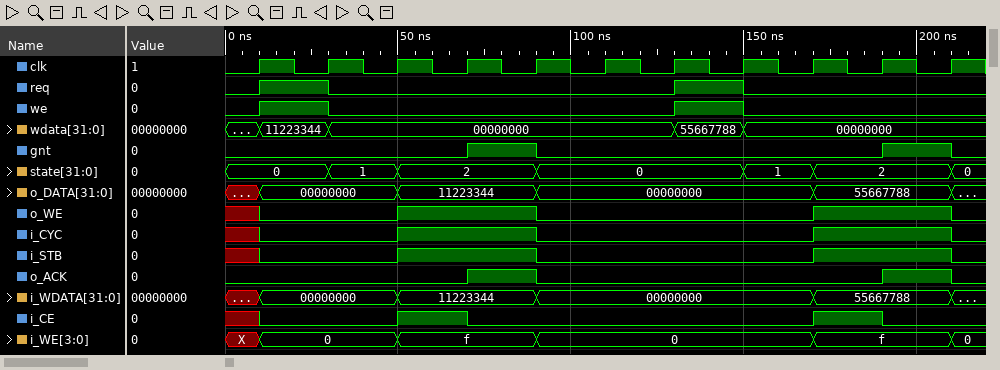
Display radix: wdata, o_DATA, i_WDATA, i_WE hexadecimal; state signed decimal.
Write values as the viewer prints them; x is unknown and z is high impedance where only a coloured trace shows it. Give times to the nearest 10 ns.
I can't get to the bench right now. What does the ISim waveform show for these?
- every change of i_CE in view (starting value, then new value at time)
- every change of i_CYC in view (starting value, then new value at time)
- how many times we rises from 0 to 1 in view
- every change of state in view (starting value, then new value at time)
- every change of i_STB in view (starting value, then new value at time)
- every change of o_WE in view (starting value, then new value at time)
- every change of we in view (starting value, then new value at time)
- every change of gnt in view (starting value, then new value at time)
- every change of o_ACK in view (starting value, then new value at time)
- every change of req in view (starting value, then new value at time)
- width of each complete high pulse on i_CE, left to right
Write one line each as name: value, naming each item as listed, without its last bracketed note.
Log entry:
every change of i_CE in view: x, 0 at 10 ns, 1 at 50 ns, 0 at 70 ns, 1 at 170 ns, 0 at 190 ns
every change of i_CYC in view: x, 0 at 10 ns, 1 at 50 ns, 0 at 90 ns, 1 at 170 ns, 0 at 210 ns
how many times we rises from 0 to 1 in view: 2
every change of state in view: 0, 1 at 30 ns, 2 at 50 ns, 0 at 90 ns, 1 at 150 ns, 2 at 170 ns, 0 at 210 ns
every change of i_STB in view: x, 0 at 10 ns, 1 at 50 ns, 0 at 90 ns, 1 at 170 ns, 0 at 210 ns
every change of o_WE in view: x, 0 at 10 ns, 1 at 50 ns, 0 at 90 ns, 1 at 170 ns, 0 at 210 ns
every change of we in view: 0, 1 at 10 ns, 0 at 30 ns, 1 at 130 ns, 0 at 150 ns
every change of gnt in view: 0, 1 at 70 ns, 0 at 90 ns, 1 at 190 ns, 0 at 210 ns
every change of o_ACK in view: 0, 1 at 70 ns, 0 at 90 ns, 1 at 190 ns, 0 at 210 ns
every change of req in view: 0, 1 at 10 ns, 0 at 30 ns, 1 at 130 ns, 0 at 150 ns
width of each complete high pulse on i_CE, left to right: 20 ns, 20 ns
